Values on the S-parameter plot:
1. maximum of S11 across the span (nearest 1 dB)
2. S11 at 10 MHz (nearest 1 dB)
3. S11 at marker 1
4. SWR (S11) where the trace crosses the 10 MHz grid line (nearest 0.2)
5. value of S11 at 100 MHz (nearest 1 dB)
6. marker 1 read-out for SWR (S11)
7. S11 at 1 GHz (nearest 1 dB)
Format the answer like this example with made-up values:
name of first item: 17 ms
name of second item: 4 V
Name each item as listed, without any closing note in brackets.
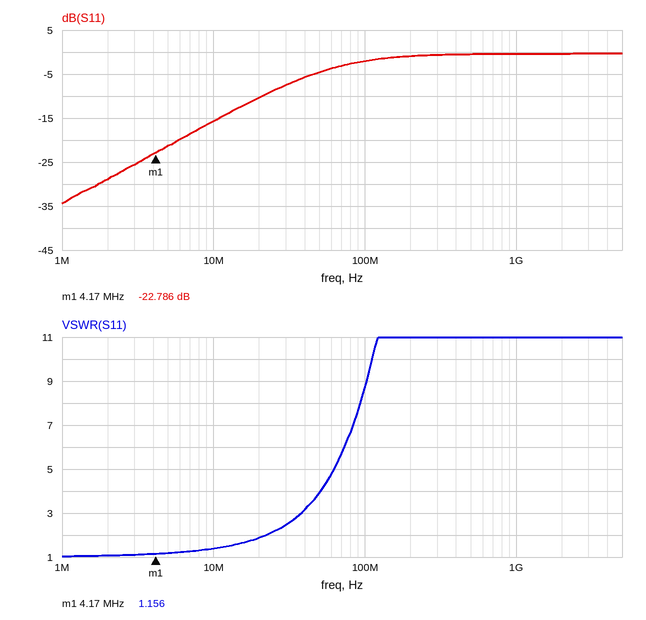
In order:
maximum of S11 across the span: 0 dB
S11 at 10 MHz: -16 dB
S11 at marker 1: -22.786 dB
SWR (S11) where the trace crosses the 10 MHz grid line: 1.4
value of S11 at 100 MHz: -2 dB
marker 1 read-out for SWR: 1.156
S11 at 1 GHz: 0 dB
